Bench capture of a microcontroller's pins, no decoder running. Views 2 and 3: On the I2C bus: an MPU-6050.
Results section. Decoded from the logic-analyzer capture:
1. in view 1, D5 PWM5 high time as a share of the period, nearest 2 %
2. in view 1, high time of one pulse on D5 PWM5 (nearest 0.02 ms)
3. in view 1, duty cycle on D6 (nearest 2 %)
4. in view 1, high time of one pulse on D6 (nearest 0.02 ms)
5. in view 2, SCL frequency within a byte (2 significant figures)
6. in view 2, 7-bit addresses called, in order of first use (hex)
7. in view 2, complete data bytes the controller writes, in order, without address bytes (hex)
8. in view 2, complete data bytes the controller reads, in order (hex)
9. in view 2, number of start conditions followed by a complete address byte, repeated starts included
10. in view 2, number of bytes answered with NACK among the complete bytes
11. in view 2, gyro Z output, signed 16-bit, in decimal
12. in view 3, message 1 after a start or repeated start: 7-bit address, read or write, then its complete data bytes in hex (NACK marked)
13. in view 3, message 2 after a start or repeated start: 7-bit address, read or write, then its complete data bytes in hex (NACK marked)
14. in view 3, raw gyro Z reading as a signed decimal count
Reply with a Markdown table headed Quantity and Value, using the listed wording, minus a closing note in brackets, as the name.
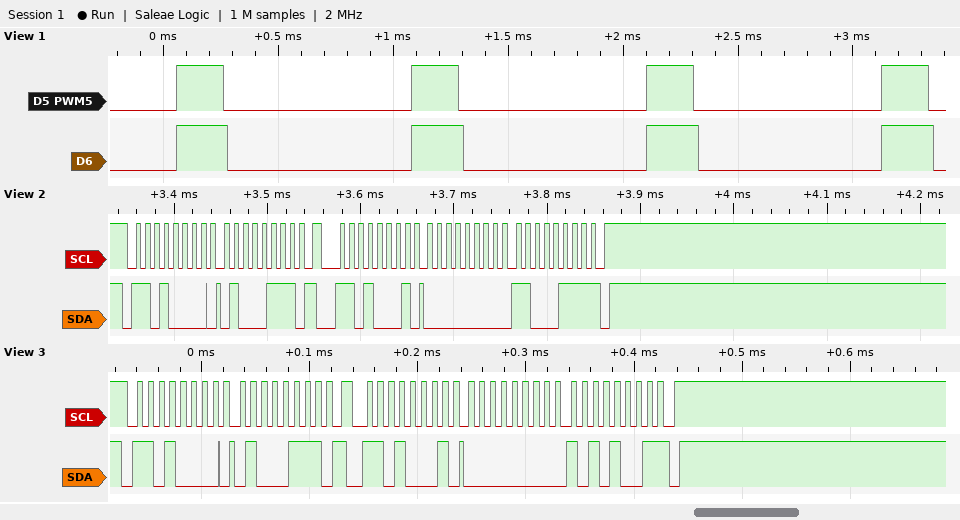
| Quantity | Value |
|---|---|
| in view 1, D5 PWM5 high time as a share of the period, nearest 2 % | 20 % |
| in view 1, high time of one pulse on D5 PWM5 | 0.20 ms |
| in view 1, duty cycle on D6 | 22 % |
| in view 1, high time of one pulse on D6 | 0.22 ms |
| in view 2, SCL frequency within a byte | 100 kHz |
| in view 2, 7-bit addresses called, in order of first use | 0x68 |
| in view 2, complete data bytes the controller writes, in order, without address bytes | 47 |
| in view 2, complete data bytes the controller reads, in order | 00 C7 |
| in view 2, number of start conditions followed by a complete address byte, repeated starts included | 2 |
| in view 2, number of bytes answered with NACK among the complete bytes | 1 |
| in view 2, gyro Z output, signed 16-bit, in decimal | 199 |
| in view 3, message 1 after a start or repeated start: 7-bit address, read or write, then its complete data bytes in hex | 0x68 write: 47 |
| in view 3, message 2 after a start or repeated start: 7-bit address, read or write, then its complete data bytes in hex | 0x68 read: 00 A9 NACK |
| in view 3, raw gyro Z reading as a signed decimal count | 169 |
